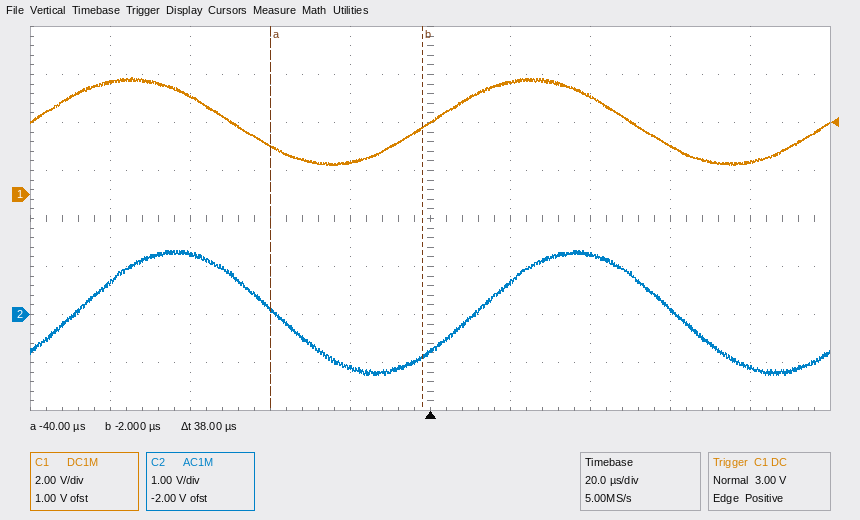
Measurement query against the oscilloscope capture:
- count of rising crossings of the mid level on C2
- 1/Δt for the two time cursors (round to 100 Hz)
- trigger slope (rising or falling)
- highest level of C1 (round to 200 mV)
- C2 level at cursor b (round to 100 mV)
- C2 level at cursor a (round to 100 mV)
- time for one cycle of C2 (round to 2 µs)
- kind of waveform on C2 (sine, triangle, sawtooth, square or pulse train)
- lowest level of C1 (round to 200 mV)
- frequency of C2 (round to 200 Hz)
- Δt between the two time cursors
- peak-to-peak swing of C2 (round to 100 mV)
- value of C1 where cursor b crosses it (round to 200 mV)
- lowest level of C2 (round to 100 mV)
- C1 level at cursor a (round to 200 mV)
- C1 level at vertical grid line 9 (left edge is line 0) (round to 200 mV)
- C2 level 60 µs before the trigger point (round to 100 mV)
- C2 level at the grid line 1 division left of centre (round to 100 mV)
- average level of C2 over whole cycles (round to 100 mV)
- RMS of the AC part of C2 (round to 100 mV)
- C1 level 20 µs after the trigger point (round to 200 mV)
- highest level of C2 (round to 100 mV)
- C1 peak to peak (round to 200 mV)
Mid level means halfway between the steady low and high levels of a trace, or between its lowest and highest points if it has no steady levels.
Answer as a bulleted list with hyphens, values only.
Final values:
- 2
- 26.3 kHz
- rising
- 4.8 V
- -900 mV
- 100 mV
- 100 µs
- sine
- 1.2 V
- 10.0 kHz
- 38 µs
- 2.6 V
- 2.8 V
- -1.3 V
- 2.0 V
- 1.4 V
- 1.3 V
- -1.1 V
- 0.0 V
- 900 mV
- 4.6 V
- 1.3 V
- 3.6 V
